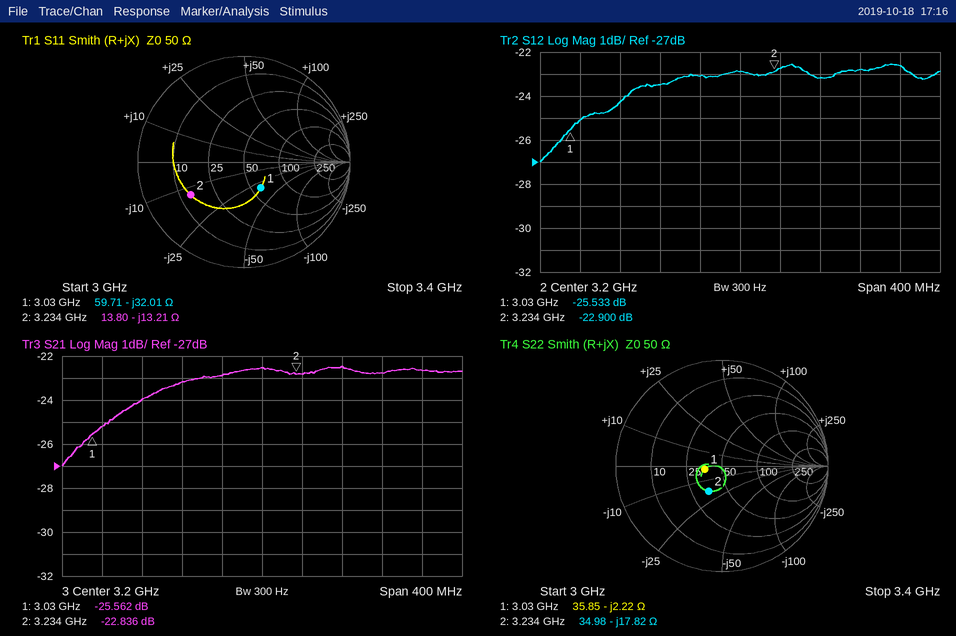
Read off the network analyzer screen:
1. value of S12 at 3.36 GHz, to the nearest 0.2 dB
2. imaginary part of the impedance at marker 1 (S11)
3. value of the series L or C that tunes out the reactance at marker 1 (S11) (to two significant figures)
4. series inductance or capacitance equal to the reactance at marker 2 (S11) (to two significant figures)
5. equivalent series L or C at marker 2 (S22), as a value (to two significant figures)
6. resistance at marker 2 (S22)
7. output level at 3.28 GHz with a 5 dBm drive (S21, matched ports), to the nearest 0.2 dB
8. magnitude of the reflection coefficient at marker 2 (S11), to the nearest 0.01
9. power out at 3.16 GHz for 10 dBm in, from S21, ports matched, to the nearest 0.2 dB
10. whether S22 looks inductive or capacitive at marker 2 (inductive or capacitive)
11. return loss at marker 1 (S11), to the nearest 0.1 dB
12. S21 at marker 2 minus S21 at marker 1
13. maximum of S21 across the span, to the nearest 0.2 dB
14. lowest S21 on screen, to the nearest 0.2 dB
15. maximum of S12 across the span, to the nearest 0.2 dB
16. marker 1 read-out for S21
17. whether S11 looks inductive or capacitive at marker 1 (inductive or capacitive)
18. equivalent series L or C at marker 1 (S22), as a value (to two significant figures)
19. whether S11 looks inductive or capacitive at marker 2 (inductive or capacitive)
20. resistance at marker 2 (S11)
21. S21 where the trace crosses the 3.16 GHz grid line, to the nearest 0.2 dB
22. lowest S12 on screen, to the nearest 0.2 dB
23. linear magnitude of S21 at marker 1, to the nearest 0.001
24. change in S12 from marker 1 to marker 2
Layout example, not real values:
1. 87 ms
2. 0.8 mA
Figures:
1. -22.6 dB
2. -32.01 Ω
3. 1.7 nH
4. 3.7 pF
5. 2.8 pF
6. 34.98 Ω
7. -17.4 dBm
8. 0.59
9. -12.8 dBm
10. capacitive
11. 10.7 dB
12. 2.726 dB
13. -22.4 dB
14. -27.0 dB
15. -22.6 dB
16. -25.562 dB
17. capacitive
18. 24 pF
19. capacitive
20. 13.80 Ω
21. -22.8 dB
22. -27.0 dB
23. 0.053
24. 2.633 dB
